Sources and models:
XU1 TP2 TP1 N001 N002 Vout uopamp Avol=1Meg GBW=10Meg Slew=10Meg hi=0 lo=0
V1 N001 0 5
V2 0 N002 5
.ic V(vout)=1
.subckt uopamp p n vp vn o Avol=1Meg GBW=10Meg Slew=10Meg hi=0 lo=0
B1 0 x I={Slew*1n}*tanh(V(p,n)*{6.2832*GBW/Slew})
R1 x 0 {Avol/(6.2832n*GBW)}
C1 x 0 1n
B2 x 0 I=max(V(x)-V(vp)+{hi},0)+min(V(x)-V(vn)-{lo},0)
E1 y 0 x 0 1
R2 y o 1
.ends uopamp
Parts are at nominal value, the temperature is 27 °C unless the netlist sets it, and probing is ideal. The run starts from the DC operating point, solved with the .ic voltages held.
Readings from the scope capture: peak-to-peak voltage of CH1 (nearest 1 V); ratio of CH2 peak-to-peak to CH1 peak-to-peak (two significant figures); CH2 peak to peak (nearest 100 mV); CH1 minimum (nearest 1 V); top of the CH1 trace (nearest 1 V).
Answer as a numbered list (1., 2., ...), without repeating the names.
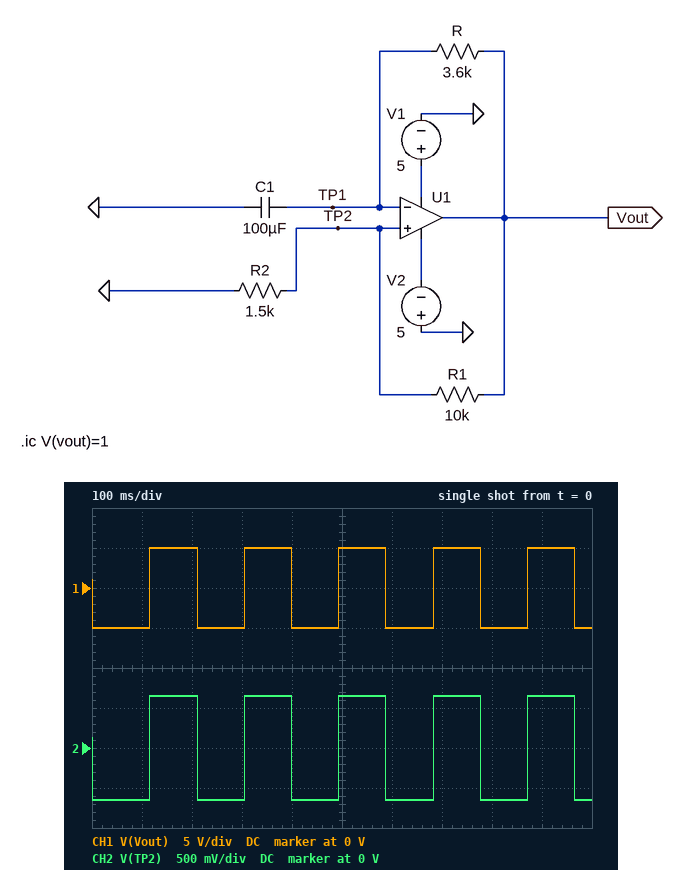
1. 10 V
2. 0.13
3. 1.3 V
4. -5 V
5. 5 V
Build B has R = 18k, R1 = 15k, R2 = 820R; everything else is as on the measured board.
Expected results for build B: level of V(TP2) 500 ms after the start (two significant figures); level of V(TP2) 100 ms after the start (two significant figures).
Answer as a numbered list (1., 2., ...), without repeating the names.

1. 260 mV
2. -260 mV
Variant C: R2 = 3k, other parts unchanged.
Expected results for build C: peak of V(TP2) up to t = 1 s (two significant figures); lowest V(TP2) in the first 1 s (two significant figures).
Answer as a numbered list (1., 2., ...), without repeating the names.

1. 1.2 V
2. -1.2 V
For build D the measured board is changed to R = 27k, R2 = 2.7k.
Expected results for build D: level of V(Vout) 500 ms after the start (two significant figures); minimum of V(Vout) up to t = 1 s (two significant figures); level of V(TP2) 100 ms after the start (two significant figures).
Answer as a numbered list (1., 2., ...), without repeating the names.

1. -5.0 V
2. -5.0 V
3. -1.1 V
